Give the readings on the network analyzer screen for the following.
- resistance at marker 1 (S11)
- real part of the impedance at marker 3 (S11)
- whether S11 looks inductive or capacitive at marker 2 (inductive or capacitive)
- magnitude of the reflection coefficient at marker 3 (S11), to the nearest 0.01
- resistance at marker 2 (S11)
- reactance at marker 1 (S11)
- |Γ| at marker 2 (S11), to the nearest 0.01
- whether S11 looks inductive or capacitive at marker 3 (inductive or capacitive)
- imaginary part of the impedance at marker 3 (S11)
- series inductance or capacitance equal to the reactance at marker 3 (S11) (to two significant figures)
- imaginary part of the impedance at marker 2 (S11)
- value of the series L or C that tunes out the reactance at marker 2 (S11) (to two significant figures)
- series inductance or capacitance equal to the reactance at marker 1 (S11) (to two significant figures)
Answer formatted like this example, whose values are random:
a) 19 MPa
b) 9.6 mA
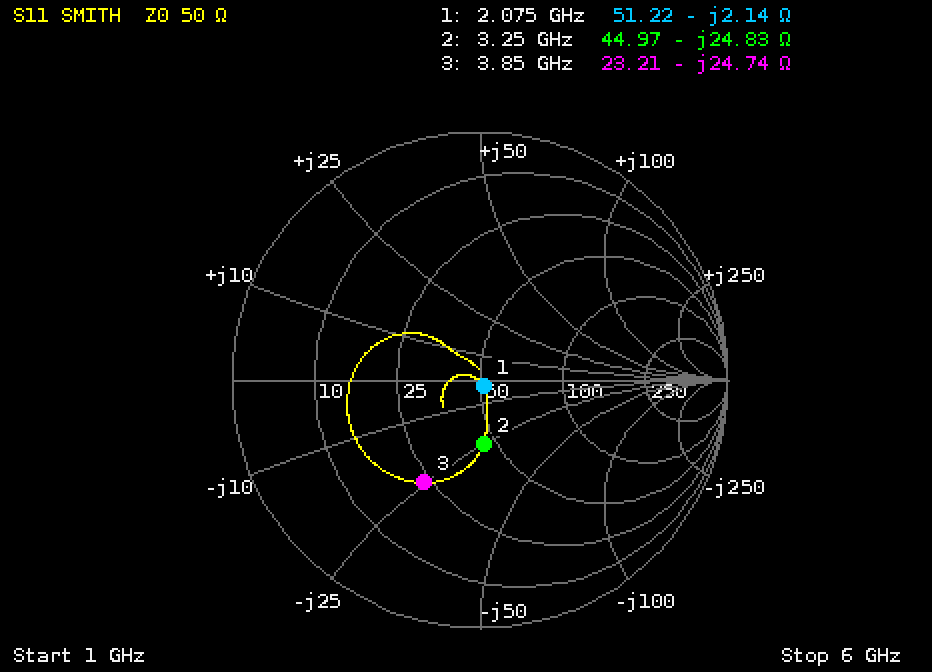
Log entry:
a) 51.22 Ω
b) 23.21 Ω
c) capacitive
d) 0.47
e) 44.97 Ω
f) -2.14 Ω
g) 0.26
h) capacitive
i) -24.74 Ω
j) 1.7 pF
k) -24.83 Ω
l) 1.2 nH
m) 36 pF
